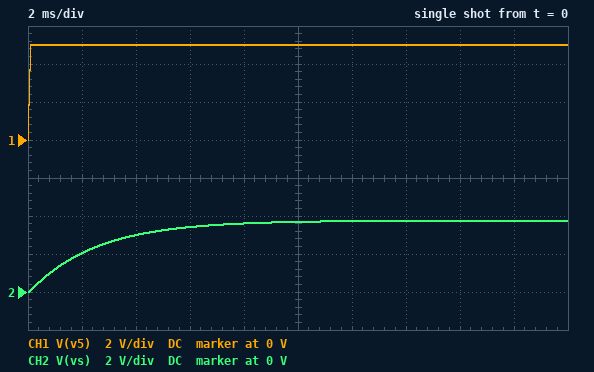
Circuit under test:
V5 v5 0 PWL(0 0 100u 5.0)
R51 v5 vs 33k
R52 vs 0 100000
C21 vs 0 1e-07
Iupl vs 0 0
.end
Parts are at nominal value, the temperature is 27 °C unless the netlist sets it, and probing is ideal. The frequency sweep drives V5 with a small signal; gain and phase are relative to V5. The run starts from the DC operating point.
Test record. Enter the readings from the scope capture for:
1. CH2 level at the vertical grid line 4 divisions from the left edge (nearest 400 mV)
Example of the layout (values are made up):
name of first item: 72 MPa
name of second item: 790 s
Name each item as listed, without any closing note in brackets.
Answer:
CH2 level at the vertical grid line 4 divisions from the left edge: 3.6 V
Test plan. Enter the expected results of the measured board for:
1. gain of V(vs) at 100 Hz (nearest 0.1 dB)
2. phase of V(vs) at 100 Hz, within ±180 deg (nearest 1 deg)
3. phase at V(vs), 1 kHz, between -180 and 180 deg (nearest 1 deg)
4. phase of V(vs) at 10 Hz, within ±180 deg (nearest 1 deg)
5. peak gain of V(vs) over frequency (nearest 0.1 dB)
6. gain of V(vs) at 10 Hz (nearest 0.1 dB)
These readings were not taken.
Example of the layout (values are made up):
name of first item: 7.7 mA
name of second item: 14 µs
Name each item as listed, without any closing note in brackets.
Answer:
gain of V(vs) at 100 Hz: -7.8 dB
phase of V(vs) at 100 Hz, within ±180 deg: -57 deg
phase at V(vs), 1 kHz, between -180 and 180 deg: -86 deg
phase of V(vs) at 10 Hz, within ±180 deg: -9 deg
peak gain of V(vs) over frequency: -2.5 dB
gain of V(vs) at 10 Hz: -2.6 dB
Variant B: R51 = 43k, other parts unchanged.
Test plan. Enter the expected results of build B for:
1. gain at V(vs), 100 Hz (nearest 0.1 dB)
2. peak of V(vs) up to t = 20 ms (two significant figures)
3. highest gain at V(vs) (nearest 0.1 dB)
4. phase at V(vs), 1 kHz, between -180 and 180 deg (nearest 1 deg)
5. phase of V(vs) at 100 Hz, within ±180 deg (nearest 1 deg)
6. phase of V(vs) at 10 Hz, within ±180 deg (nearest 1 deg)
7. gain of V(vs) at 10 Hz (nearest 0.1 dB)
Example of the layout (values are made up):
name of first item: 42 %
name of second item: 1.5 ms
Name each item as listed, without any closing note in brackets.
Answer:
gain at V(vs), 100 Hz: -9.7 dB
peak of V(vs) up to t = 20 ms: 3.5 V
highest gain at V(vs): -3.1 dB
phase at V(vs), 1 kHz, between -180 and 180 deg: -87 deg
phase of V(vs) at 100 Hz, within ±180 deg: -62 deg
phase of V(vs) at 10 Hz, within ±180 deg: -11 deg
gain of V(vs) at 10 Hz: -3.3 dB
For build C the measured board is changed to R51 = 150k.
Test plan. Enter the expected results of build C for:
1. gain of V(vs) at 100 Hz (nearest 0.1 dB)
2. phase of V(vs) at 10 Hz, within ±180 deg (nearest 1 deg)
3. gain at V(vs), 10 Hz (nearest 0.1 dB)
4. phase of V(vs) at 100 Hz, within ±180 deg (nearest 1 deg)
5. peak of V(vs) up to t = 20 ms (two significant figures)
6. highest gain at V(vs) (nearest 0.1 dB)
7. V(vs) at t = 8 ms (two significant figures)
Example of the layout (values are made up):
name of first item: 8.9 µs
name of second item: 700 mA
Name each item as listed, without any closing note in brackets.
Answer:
gain of V(vs) at 100 Hz: -19.8 dB
phase of V(vs) at 10 Hz, within ±180 deg: -21 deg
gain at V(vs), 10 Hz: -8.5 dB
phase of V(vs) at 100 Hz, within ±180 deg: -75 deg
peak of V(vs) up to t = 20 ms: 1.9 V
highest gain at V(vs): -8.0 dB
V(vs) at t = 8 ms: 1.5 V
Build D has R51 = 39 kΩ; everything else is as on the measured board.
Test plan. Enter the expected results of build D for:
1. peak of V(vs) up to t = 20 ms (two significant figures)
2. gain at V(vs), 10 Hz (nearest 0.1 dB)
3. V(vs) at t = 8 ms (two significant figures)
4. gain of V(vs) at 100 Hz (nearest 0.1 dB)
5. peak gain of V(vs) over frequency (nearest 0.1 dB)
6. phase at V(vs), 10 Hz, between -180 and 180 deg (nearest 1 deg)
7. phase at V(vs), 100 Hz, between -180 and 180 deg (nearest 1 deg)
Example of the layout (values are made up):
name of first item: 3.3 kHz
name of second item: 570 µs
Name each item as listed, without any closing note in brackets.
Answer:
peak of V(vs) up to t = 20 ms: 3.6 V
gain at V(vs), 10 Hz: -3.0 dB
V(vs) at t = 8 ms: 3.4 V
gain of V(vs) at 100 Hz: -9.0 dB
peak gain of V(vs) over frequency: -2.9 dB
phase at V(vs), 10 Hz, between -180 and 180 deg: -10 deg
phase at V(vs), 100 Hz, between -180 and 180 deg: -60 deg
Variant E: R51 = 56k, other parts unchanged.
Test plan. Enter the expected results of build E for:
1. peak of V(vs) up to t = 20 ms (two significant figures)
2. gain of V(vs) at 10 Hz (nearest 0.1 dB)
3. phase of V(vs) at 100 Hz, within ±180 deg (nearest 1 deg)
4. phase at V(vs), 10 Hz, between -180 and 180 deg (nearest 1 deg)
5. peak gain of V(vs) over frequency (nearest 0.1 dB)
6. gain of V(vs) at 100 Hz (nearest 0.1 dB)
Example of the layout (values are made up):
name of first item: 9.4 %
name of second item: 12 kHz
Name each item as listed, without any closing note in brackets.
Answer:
peak of V(vs) up to t = 20 ms: 3.2 V
gain of V(vs) at 10 Hz: -4.1 dB
phase of V(vs) at 100 Hz, within ±180 deg: -66 deg
phase at V(vs), 10 Hz, between -180 and 180 deg: -13 deg
peak gain of V(vs) over frequency: -3.9 dB
gain of V(vs) at 100 Hz: -11.7 dB
